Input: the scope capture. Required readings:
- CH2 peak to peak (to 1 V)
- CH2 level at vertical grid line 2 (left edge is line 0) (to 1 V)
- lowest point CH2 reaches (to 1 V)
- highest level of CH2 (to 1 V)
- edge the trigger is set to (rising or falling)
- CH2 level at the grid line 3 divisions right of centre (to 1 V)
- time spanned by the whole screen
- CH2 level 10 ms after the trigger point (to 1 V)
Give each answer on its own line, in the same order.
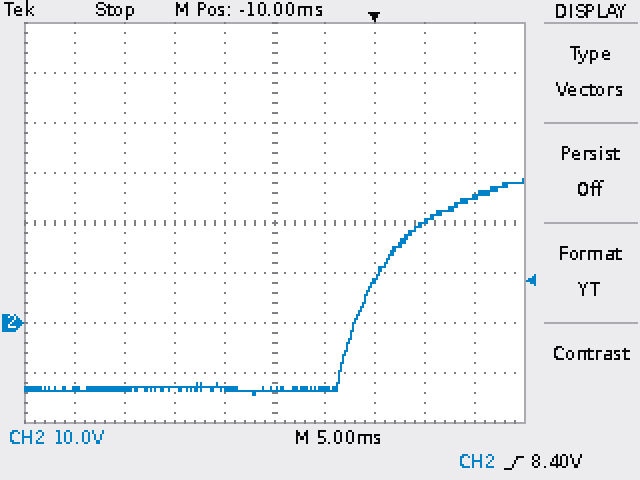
43 V
-13 V
-14 V
29 V
rising
20 V
50 ms
25 V
